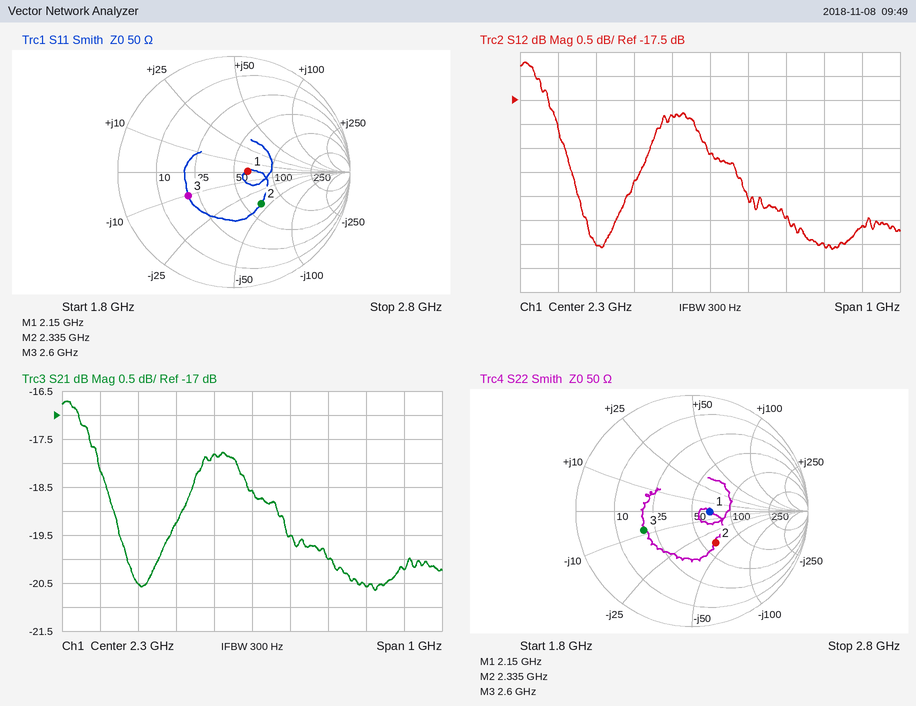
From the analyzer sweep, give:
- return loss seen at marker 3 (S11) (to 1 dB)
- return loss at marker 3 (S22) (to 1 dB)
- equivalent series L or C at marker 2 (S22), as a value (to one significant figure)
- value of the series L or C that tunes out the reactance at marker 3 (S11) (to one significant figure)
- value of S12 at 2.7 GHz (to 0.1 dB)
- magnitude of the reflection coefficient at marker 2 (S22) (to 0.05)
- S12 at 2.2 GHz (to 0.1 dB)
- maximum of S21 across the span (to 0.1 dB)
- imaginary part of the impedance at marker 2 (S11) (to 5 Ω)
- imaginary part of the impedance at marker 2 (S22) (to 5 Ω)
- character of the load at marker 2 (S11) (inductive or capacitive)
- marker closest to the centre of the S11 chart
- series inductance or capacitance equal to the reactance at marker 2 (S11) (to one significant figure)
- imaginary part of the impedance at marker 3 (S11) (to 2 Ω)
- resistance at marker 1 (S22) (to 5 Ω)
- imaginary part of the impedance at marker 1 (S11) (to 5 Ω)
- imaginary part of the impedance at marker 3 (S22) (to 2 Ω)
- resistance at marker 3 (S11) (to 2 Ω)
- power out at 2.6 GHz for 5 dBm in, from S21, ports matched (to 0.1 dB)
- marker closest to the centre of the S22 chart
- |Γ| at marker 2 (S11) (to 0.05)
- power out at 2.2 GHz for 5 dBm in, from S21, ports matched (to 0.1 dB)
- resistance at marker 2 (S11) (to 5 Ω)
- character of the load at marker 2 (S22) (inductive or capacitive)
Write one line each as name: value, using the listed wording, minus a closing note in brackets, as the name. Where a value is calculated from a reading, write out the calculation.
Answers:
return loss seen at marker 3 (S11): 7 dB
return loss at marker 3 (S22): 7 dB
equivalent series L or C at marker 2 (S22), as a value: C = 1/(2π × 2.335 GHz × 40 Ω) ≈ 2 pF
value of the series L or C that tunes out the reactance at marker 3 (S11): L = 10 Ω/(2π × 2.6 GHz) ≈ 612 pH, so 600 pH to one significant figure
value of S12 at 2.7 GHz: -20.1 dB
magnitude of the reflection coefficient at marker 2 (S22): 0.35
S12 at 2.2 GHz: -17.8 dB
maximum of S21 across the span: -16.7 dB
imaginary part of the impedance at marker 2 (S11): -40 Ω
imaginary part of the impedance at marker 2 (S22): -40 Ω
character of the load at marker 2 (S11): capacitive
marker closest to the centre of the S11 chart: marker 1
series inductance or capacitance equal to the reactance at marker 2 (S11): C = 1/(2π × 2.335 GHz × 40 Ω) ≈ 2 pF
imaginary part of the impedance at marker 3 (S11): -10 Ω
resistance at marker 1 (S22): 70 Ω
imaginary part of the impedance at marker 1 (S11): 0 Ω
imaginary part of the impedance at marker 3 (S22): -8 Ω
resistance at marker 3 (S11): 20 Ω
power out at 2.6 GHz for 5 dBm in, from S21, ports matched: 5 dBm + (-20.6 dB) = -15.6 dBm
marker closest to the centre of the S22 chart: marker 1
|Γ| at marker 2 (S11): 0.35
power out at 2.2 GHz for 5 dBm in, from S21, ports matched: 5 dBm + (-17.8 dB) = -12.8 dBm
resistance at marker 2 (S11): 65 Ω
character of the load at marker 2 (S22): capacitive
